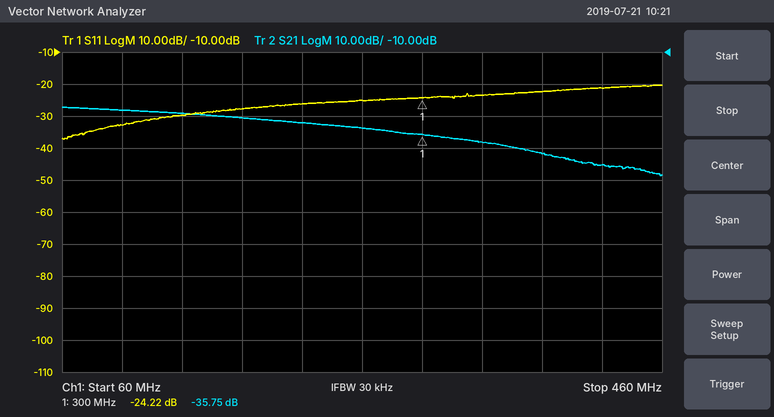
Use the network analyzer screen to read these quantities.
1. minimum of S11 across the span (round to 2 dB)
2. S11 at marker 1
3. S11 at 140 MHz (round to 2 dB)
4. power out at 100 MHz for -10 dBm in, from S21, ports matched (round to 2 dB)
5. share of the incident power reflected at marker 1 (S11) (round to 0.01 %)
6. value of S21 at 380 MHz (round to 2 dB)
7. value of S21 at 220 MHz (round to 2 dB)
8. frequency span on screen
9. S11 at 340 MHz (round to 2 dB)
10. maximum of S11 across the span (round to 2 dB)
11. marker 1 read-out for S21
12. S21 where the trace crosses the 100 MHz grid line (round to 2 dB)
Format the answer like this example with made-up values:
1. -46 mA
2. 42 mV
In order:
1. -38 dB
2. -24.22 dB
3. -30 dB
4. -38 dBm
5. 0.38 %
6. -42 dB
7. -32 dB
8. 400 MHz
9. -24 dB
10. -20 dB
11. -35.75 dB
12. -28 dB
